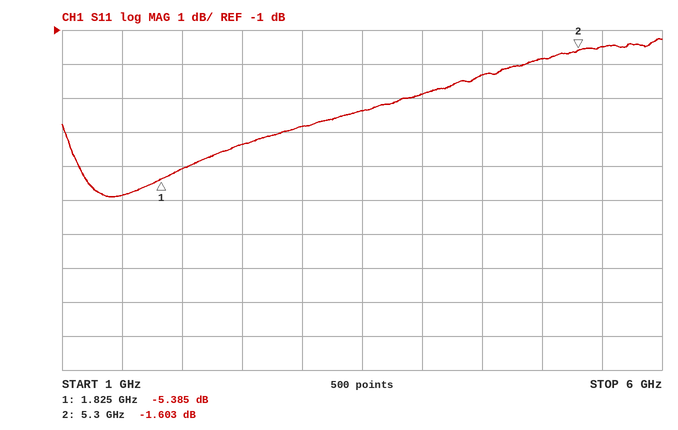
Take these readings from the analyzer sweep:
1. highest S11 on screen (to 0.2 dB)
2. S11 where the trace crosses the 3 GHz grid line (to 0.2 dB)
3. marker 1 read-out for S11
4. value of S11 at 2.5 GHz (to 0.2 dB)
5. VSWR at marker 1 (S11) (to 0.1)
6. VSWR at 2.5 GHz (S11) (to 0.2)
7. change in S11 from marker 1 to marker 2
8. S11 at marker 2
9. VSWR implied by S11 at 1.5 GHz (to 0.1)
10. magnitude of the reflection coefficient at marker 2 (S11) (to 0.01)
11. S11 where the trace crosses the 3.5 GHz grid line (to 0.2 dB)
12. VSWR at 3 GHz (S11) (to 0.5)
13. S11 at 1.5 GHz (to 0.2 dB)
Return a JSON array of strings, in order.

["-1.2 dB", "-3.8 dB", "-5.385 dB", "-4.4 dB", "3.3", "4.0", "3.782 dB", "-1.603 dB", "3.1", "0.83", "-3.4 dB", "4.5", "-5.8 dB"]
